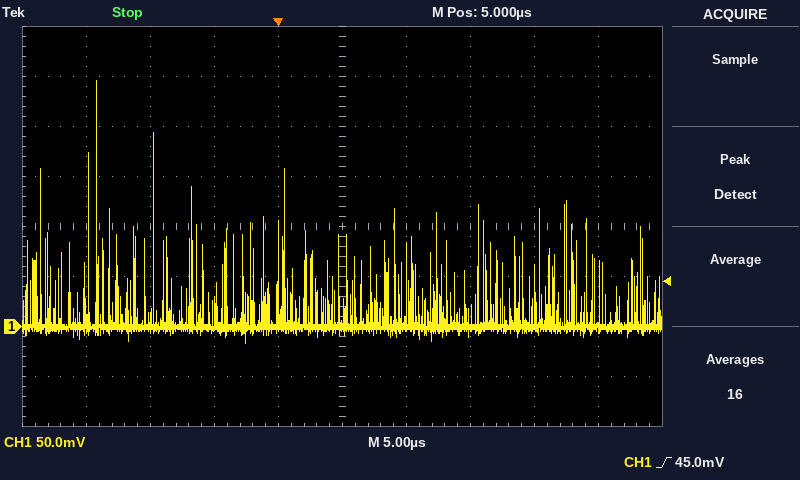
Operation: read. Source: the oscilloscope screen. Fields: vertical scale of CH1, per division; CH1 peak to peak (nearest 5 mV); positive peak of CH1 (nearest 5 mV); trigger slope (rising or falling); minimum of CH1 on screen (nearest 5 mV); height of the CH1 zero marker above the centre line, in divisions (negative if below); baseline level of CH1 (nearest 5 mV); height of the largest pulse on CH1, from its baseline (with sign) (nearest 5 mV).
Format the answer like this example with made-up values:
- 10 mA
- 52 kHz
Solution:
- 50 mV
- 260 mV
- 245 mV
- rising
- -15 mV
- -2.0 div
- 0 mV
- +245 mV
